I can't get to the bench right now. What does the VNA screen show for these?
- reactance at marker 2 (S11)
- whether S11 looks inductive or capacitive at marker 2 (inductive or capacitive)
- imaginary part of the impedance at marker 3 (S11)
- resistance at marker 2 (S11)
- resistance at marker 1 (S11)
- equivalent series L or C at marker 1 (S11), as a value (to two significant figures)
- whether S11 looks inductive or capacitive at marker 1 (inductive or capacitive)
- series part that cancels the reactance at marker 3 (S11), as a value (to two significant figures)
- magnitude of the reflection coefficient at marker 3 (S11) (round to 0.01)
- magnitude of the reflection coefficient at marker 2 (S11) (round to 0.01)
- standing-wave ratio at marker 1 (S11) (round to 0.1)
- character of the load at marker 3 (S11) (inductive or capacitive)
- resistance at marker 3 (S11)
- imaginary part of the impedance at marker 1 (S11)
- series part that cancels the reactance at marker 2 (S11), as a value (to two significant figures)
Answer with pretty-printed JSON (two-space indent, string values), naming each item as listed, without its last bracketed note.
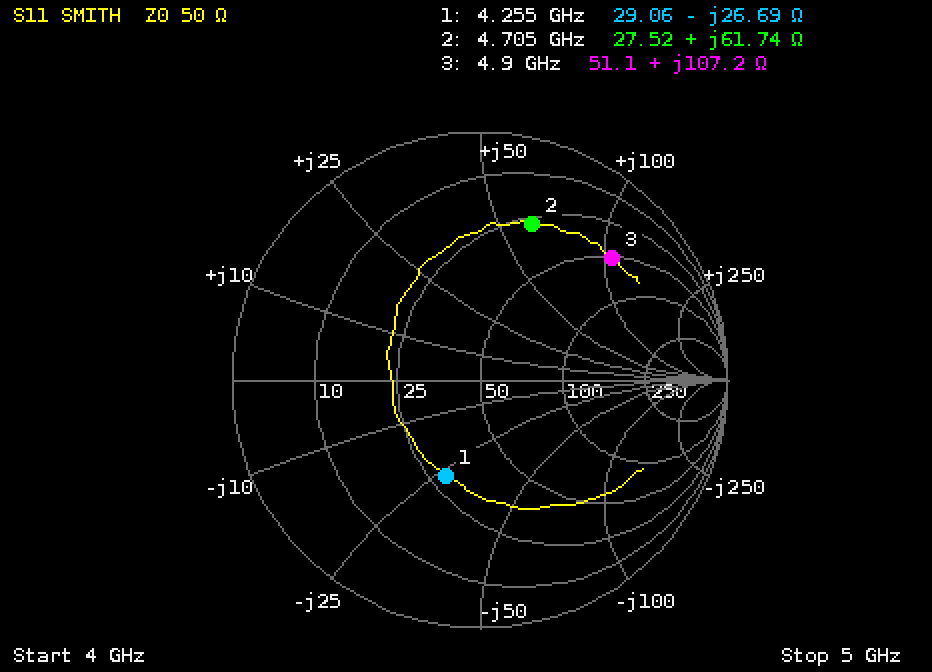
{
  "reactance at marker 2": "+61.74 Ω",
  "whether S11 looks inductive or capacitive at marker 2": "inductive",
  "imaginary part of the impedance at marker 3": "+107.2 Ω",
  "resistance at marker 2": "27.52 Ω",
  "resistance at marker 1": "29.06 Ω",
  "equivalent series L or C at marker 1 (S11), as a value": "1.4 pF",
  "whether S11 looks inductive or capacitive at marker 1": "capacitive",
  "series part that cancels the reactance at marker 3 (S11), as a value": "300 fF",
  "magnitude of the reflection coefficient at marker 3 (S11)": "0.73",
  "magnitude of the reflection coefficient at marker 2 (S11)": "0.66",
  "standing-wave ratio at marker 1 (S11)": "2.4",
  "character of the load at marker 3 (S11)": "inductive",
  "resistance at marker 3": "51.1 Ω",
  "imaginary part of the impedance at marker 1": "-26.69 Ω",
  "series part that cancels the reactance at marker 2 (S11), as a value": "550 fF"
}
